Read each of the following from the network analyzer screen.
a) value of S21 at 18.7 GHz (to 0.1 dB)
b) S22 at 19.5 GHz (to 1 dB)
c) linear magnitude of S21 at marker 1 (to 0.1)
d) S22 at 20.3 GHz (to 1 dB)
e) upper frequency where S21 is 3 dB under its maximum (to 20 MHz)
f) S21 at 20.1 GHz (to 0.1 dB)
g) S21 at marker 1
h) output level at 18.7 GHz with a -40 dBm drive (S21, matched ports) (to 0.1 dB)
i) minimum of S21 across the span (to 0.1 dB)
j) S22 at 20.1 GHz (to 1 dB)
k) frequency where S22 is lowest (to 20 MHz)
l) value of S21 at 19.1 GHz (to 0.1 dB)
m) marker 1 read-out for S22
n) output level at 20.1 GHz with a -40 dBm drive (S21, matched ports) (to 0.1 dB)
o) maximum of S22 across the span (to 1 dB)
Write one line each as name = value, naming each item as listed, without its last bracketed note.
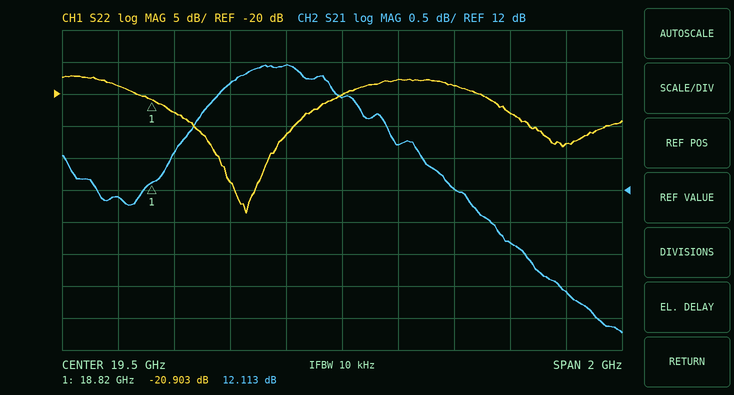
value of S21 at 18.7 GHz = 11.9 dB
S22 at 19.5 GHz = -20 dB
linear magnitude of S21 at marker 1 = 4.0
S22 at 20.3 GHz = -28 dB
upper frequency where S21 is 3 dB under its maximum = 20.16 GHz
S21 at 20.1 GHz = 11.2 dB
S21 at marker 1 = 12.113 dB
output level at 18.7 GHz with a -40 dBm drive (S21, matched ports) = -28.1 dBm
minimum of S21 across the span = 9.8 dB
S22 at 20.1 GHz = -23 dB
frequency where S22 is lowest = 19.16 GHz
value of S21 at 19.1 GHz = 13.7 dB
marker 1 read-out for S22 = -20.903 dB
output level at 20.1 GHz with a -40 dBm drive (S21, matched ports) = -28.8 dBm
maximum of S22 across the span = -17 dB
